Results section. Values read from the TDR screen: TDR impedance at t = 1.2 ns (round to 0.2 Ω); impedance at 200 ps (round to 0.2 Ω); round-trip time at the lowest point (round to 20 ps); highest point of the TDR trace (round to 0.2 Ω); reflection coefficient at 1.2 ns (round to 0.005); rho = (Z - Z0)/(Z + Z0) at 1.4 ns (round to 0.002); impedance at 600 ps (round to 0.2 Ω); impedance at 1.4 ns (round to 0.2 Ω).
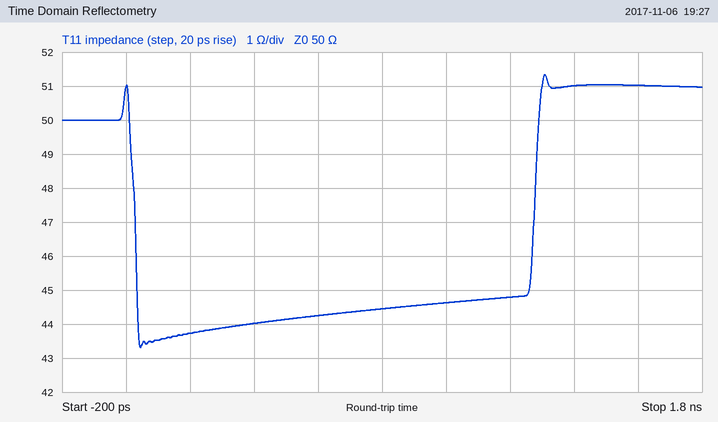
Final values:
44.8 Ω
43.8 Ω
40 ps
51.4 Ω
-0.055
+0.010
44.2 Ω
51.0 Ω
